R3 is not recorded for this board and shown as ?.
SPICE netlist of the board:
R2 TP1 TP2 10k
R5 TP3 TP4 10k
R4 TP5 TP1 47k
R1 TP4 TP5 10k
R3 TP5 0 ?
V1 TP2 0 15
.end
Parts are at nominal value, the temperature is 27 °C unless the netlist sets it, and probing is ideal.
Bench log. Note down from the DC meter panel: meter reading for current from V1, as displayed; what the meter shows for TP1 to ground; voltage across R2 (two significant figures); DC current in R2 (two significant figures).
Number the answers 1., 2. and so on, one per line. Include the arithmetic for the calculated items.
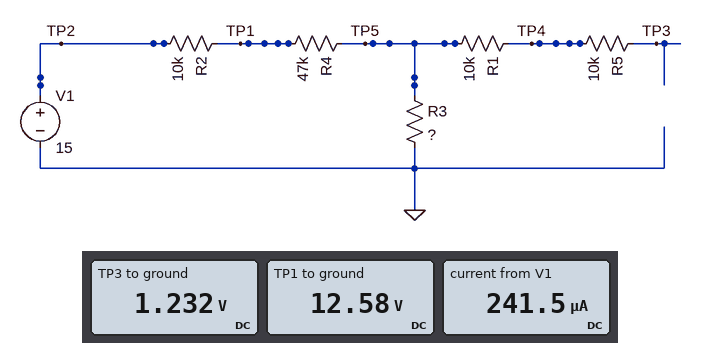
1. 241.5 µA
2. 12.58 V
3. 15 V - 12.58 V = 2.4 V
4. (15 V - 12.58 V) / 10 kΩ = 240 µA
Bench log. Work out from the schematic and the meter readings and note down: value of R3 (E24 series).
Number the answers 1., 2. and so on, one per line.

1. 5.1 kΩ
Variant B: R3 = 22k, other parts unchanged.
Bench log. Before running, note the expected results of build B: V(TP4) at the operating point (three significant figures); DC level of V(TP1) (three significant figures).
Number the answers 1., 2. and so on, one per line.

1. 4.18 V
2. 13.1 V
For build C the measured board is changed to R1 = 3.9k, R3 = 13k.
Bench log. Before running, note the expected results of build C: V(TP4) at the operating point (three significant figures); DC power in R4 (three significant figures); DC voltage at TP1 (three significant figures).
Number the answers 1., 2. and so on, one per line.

1. 2.79 V
2. 2.16 mW
3. 12.9 V
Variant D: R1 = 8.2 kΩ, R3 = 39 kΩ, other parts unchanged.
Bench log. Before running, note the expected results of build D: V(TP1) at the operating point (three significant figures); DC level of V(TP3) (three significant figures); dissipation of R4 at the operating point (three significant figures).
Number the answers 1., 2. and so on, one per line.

1. 13.4 V
2. 6.09 V
3. 1.15 mW
